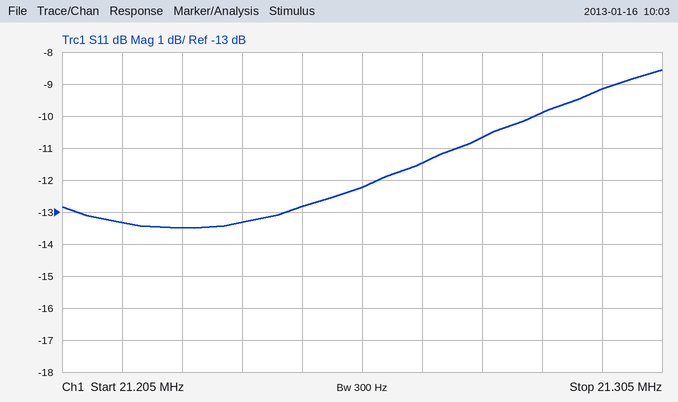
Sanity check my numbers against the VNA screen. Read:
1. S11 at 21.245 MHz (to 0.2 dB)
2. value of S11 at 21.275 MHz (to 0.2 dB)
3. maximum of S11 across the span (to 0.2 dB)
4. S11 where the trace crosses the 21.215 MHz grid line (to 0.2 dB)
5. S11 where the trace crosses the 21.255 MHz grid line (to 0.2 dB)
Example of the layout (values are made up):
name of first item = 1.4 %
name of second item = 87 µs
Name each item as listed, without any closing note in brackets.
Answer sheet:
S11 at 21.245 MHz = -12.8 dB
value of S11 at 21.275 MHz = -10.6 dB
maximum of S11 across the span = -8.6 dB
S11 where the trace crosses the 21.215 MHz grid line = -13.4 dB
S11 where the trace crosses the 21.255 MHz grid line = -12.2 dB
